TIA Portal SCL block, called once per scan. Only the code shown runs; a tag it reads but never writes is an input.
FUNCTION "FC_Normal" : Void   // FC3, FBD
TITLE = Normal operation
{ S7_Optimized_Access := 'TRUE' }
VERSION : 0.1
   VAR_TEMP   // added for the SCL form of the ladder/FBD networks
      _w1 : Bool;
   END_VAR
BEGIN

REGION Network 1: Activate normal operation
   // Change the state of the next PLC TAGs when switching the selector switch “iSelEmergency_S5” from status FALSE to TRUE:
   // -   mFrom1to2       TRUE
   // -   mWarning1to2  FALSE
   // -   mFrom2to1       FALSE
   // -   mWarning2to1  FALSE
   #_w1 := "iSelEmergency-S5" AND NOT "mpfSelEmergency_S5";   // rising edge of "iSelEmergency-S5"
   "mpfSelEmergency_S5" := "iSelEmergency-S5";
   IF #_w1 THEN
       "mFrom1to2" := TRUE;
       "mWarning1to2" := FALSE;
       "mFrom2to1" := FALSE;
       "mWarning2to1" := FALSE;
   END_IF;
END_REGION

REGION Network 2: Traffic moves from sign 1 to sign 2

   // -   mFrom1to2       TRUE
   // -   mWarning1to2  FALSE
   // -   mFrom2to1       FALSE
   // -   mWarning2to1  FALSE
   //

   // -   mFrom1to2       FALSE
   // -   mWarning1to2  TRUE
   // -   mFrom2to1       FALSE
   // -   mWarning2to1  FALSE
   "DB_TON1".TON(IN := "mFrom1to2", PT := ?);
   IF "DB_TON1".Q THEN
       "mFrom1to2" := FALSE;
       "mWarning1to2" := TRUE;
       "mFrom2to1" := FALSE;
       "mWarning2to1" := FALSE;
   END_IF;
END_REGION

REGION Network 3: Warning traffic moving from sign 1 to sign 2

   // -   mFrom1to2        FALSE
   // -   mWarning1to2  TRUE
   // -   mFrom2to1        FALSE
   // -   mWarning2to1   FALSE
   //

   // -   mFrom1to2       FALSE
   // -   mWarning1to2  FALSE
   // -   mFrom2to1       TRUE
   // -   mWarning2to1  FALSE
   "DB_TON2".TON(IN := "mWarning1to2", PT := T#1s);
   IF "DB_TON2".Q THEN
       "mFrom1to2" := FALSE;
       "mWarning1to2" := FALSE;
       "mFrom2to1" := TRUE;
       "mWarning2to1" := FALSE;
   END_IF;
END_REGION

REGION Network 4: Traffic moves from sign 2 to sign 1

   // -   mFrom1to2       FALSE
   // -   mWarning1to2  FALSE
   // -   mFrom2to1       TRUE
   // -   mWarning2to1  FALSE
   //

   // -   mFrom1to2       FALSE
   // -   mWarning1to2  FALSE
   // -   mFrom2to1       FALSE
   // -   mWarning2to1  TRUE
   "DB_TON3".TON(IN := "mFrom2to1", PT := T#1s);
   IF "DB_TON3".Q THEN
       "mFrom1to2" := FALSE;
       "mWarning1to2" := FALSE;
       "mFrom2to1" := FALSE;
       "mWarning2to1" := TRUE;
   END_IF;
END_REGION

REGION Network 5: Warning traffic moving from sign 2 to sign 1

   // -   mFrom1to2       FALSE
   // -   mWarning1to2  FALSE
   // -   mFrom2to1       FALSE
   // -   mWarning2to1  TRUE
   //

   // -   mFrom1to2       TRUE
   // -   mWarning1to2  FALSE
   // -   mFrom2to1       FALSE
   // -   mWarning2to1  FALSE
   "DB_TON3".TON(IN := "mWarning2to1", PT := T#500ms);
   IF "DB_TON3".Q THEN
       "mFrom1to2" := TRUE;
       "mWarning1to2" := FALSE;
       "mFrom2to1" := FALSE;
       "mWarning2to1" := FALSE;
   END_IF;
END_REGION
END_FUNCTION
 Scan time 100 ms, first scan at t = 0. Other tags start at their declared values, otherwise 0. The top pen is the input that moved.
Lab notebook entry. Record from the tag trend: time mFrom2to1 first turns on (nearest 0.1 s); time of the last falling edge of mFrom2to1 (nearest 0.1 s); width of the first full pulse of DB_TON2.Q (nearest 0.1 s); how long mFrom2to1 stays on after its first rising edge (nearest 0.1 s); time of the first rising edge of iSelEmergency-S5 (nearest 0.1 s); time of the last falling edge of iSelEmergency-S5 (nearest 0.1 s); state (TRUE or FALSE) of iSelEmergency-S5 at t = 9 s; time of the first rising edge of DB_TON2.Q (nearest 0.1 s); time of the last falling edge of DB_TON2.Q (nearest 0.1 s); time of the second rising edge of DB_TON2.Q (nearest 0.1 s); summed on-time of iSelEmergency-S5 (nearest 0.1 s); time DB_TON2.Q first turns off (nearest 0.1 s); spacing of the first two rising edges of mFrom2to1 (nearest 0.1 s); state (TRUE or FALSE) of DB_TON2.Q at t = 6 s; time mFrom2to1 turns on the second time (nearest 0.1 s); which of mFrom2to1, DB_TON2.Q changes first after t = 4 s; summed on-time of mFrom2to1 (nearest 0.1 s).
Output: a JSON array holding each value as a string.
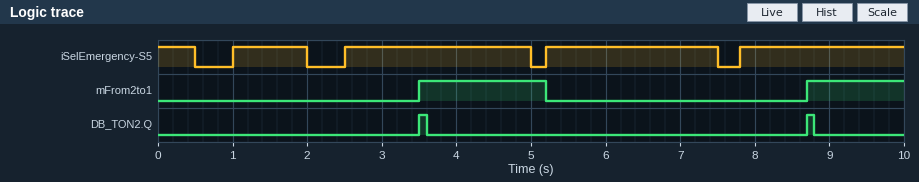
["3.5 s", "5.2 s", "0.1 s", "1.7 s", "1.0 s", "7.5 s", "TRUE", "3.5 s", "8.8 s", "8.7 s", "8.5 s", "3.6 s", "5.2 s", "FALSE", "8.7 s", "mFrom2to1", "3.0 s"]
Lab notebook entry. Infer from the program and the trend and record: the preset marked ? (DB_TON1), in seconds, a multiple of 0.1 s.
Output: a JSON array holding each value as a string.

["2.5 s"]
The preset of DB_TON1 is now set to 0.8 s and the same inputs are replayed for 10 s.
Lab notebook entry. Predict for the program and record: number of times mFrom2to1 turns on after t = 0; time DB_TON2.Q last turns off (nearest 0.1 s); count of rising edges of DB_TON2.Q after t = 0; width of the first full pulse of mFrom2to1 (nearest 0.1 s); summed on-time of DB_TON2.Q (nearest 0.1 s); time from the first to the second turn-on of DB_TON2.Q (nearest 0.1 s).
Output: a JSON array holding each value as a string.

["3", "9.7 s", "3", "0.9 s", "0.3 s", "2.7 s"]
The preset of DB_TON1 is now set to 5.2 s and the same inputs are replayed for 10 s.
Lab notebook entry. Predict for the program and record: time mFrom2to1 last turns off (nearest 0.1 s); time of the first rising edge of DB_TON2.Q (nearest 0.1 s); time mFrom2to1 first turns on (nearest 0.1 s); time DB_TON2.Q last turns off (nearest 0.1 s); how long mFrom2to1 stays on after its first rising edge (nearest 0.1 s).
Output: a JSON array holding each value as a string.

["7.8 s", "6.2 s", "6.2 s", "6.3 s", "1.6 s"]
